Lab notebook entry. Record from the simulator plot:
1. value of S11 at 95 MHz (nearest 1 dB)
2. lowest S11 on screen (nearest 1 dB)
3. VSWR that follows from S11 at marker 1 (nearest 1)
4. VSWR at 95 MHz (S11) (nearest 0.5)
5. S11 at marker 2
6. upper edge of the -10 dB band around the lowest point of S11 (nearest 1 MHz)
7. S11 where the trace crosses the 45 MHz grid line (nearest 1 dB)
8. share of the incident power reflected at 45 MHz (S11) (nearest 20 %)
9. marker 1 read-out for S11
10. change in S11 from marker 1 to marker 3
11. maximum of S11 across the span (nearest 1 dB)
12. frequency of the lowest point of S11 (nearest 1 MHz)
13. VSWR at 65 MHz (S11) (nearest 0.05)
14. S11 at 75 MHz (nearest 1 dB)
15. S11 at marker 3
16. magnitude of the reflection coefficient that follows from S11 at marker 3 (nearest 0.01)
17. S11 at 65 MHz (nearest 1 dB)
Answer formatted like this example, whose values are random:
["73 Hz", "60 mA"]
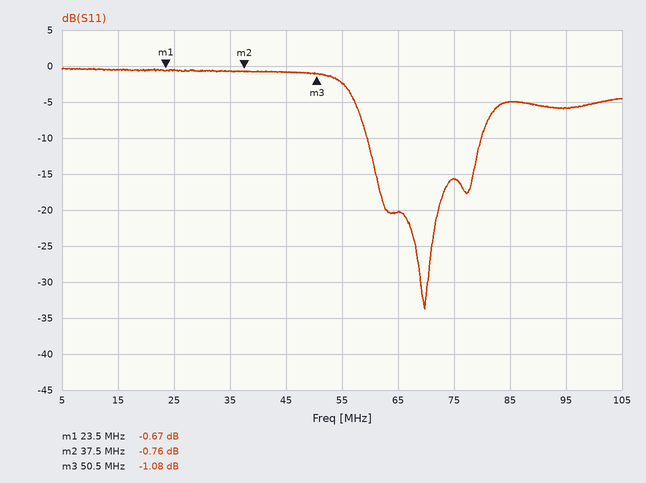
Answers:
["-6 dB", "-34 dB", "26", "3.0", "-0.76 dB", "80 MHz", "-1 dB", "80 %", "-0.67 dB", "-0.41 dB", "0 dB", "70 MHz", "1.20", "-16 dB", "-1.08 dB", "0.88", "-20 dB"]
